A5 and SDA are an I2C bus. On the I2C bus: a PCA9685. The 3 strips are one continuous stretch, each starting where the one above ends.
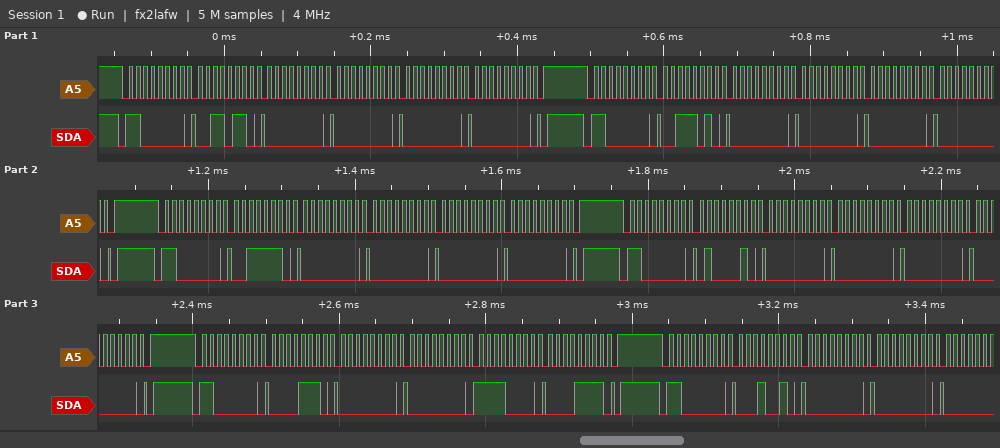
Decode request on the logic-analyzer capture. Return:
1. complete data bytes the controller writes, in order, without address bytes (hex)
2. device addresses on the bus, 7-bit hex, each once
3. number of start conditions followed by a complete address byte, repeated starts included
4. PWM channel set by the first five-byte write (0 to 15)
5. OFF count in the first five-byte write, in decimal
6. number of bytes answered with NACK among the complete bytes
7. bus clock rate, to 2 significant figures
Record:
36 00 00 00 00 3A 00 00 00 00 3E 00 00 00 00 42 00 00 00 00 0E 00 00 F0 0F 12 00 00
0x60
6
12
0
0
100 kHz
